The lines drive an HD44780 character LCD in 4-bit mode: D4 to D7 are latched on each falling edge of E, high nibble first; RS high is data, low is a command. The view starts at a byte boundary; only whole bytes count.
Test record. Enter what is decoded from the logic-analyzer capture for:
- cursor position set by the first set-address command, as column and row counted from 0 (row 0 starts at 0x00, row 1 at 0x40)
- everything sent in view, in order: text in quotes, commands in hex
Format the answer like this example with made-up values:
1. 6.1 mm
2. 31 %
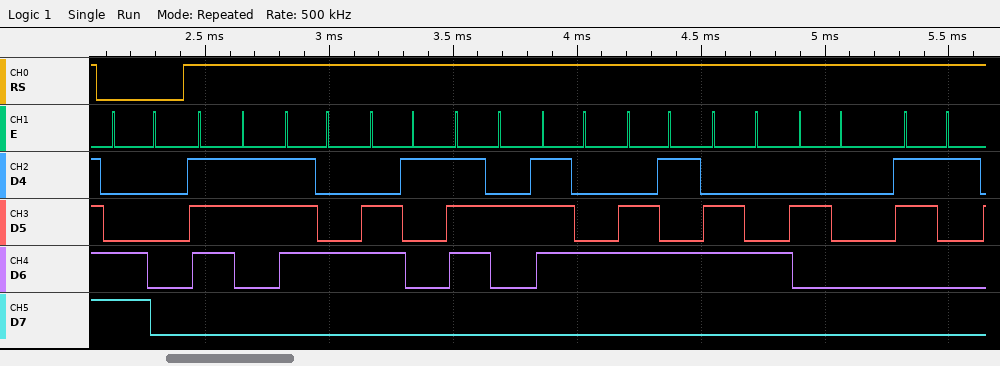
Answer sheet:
1. column 0, row 1
2. 0xC0 "started 1"
